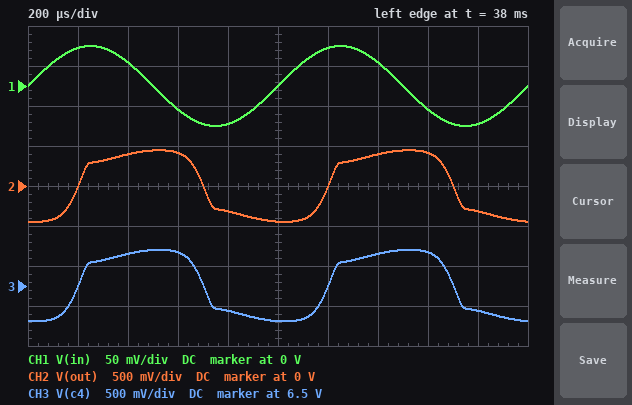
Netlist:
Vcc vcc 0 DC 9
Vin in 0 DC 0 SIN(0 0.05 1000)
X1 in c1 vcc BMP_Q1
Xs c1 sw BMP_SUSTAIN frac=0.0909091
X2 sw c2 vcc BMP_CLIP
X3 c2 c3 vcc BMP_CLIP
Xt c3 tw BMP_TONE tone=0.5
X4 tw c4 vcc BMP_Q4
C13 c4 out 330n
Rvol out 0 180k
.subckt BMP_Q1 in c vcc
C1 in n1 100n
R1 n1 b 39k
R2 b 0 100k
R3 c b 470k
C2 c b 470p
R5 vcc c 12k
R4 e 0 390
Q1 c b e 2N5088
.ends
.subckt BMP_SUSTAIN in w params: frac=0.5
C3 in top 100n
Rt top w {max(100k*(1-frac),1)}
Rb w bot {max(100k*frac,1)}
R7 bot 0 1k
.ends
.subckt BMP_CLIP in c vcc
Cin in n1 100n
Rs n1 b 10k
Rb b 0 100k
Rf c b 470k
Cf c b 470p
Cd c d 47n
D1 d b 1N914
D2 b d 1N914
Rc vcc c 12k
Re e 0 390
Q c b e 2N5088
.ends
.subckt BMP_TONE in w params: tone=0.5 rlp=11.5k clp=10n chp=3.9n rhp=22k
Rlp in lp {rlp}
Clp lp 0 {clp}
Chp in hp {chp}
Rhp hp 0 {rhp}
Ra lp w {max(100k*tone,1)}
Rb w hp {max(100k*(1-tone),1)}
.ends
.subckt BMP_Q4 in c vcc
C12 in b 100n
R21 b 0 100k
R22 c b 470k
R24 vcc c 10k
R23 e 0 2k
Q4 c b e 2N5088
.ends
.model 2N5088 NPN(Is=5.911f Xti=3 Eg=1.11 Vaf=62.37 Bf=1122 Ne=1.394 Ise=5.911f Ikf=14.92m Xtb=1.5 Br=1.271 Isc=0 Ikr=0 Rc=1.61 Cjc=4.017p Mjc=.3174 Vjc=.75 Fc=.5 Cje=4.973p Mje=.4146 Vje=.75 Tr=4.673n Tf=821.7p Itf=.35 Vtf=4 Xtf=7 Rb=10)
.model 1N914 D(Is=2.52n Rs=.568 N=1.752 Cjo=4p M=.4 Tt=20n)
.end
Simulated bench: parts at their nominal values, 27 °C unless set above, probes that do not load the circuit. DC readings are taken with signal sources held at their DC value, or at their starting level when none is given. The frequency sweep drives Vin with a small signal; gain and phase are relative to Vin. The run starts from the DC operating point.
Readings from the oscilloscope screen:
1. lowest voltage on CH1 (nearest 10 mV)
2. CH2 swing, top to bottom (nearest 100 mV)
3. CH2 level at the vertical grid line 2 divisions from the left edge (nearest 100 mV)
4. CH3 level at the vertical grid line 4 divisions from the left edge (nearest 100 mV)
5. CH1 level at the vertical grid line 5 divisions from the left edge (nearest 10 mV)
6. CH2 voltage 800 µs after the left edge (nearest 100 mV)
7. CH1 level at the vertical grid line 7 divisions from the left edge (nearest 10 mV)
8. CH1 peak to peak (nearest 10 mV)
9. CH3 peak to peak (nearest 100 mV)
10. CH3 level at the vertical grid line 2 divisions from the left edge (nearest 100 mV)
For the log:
-50 mV
900 mV
400 mV
6.2 V
0 V
-300 mV
30 mV
100 mV
900 mV
6.9 V
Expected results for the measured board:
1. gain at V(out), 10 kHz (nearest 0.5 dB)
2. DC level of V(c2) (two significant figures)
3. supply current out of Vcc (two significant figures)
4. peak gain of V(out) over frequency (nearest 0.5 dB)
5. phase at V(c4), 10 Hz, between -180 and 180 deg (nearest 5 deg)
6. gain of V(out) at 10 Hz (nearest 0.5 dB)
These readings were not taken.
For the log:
-7.5 dB
4.7 V
1.3 mA
38.5 dB
-15 deg
-10.5 dB
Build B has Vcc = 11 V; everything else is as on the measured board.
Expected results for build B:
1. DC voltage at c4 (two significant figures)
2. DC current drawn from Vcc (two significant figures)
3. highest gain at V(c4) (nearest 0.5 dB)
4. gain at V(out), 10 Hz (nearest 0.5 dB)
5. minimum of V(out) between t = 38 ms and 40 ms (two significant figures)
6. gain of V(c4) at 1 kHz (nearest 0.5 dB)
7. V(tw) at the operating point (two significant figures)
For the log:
7.6 V
1.8 mA
39.0 dB
-10.0 dB
-460 mV
32.0 dB
2.7 V
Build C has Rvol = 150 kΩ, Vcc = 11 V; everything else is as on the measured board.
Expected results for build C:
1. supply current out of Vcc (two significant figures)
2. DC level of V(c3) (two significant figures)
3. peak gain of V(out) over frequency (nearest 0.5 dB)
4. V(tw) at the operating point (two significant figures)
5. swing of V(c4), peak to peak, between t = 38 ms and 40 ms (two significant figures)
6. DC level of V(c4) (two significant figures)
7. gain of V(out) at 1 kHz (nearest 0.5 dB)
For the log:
1.8 mA
5.0 V
39.0 dB
2.7 V
910 mV
7.6 V
32.0 dB
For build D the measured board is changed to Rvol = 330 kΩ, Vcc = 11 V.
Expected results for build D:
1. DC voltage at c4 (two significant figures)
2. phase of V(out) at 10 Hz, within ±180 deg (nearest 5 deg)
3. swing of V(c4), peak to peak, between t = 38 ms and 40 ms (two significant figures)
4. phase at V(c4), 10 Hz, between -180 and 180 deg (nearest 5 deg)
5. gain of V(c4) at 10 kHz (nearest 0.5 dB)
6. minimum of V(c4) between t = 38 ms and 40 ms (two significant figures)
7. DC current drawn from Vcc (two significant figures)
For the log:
7.6 V
-5 deg
940 mV
-10 deg
-7.0 dB
7.1 V
1.8 mA
